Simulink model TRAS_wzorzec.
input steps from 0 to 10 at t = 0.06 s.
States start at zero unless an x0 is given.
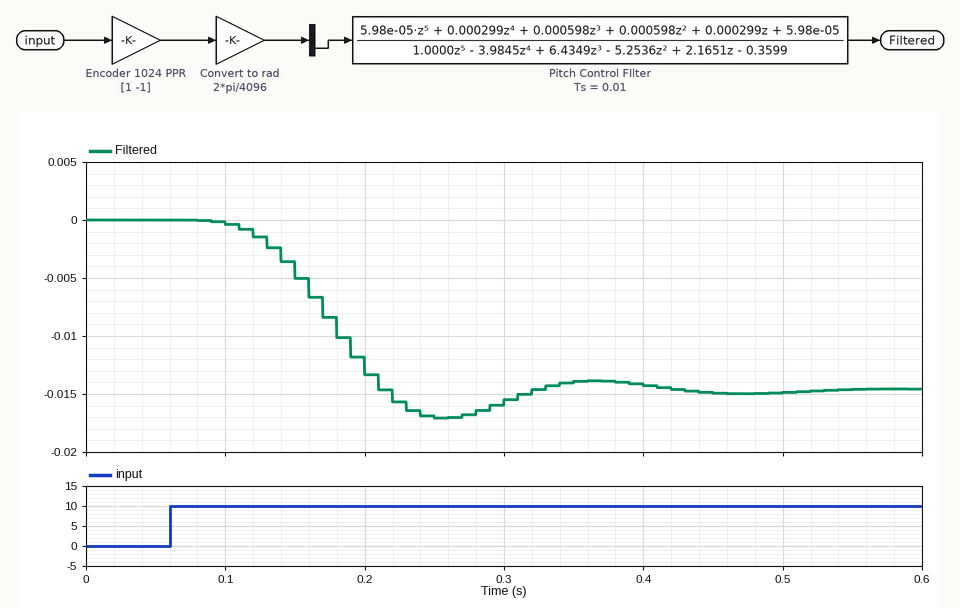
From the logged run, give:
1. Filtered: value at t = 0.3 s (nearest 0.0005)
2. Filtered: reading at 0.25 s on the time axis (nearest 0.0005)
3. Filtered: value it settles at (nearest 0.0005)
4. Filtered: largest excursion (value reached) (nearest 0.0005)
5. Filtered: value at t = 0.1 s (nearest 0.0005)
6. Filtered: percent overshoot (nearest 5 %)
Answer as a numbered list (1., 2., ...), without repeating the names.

1. -0.0155
2. -0.0170
3. -0.0145
4. -0.0170
5. -0.0005
6. 15 %
